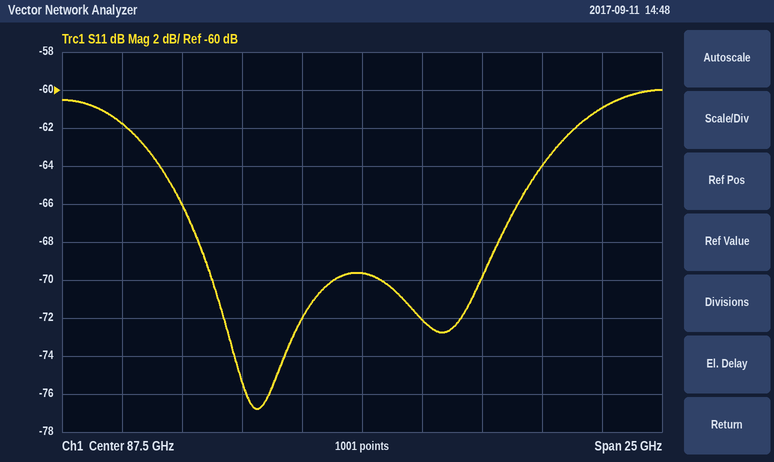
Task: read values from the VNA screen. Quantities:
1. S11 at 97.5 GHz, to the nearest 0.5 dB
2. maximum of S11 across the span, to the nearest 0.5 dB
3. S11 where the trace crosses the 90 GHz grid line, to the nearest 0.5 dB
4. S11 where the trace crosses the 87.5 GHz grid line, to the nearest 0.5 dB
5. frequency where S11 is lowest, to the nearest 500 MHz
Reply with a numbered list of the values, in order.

1. -61.0 dB
2. -60.0 dB
3. -72.0 dB
4. -69.5 dB
5. 83.0 GHz
